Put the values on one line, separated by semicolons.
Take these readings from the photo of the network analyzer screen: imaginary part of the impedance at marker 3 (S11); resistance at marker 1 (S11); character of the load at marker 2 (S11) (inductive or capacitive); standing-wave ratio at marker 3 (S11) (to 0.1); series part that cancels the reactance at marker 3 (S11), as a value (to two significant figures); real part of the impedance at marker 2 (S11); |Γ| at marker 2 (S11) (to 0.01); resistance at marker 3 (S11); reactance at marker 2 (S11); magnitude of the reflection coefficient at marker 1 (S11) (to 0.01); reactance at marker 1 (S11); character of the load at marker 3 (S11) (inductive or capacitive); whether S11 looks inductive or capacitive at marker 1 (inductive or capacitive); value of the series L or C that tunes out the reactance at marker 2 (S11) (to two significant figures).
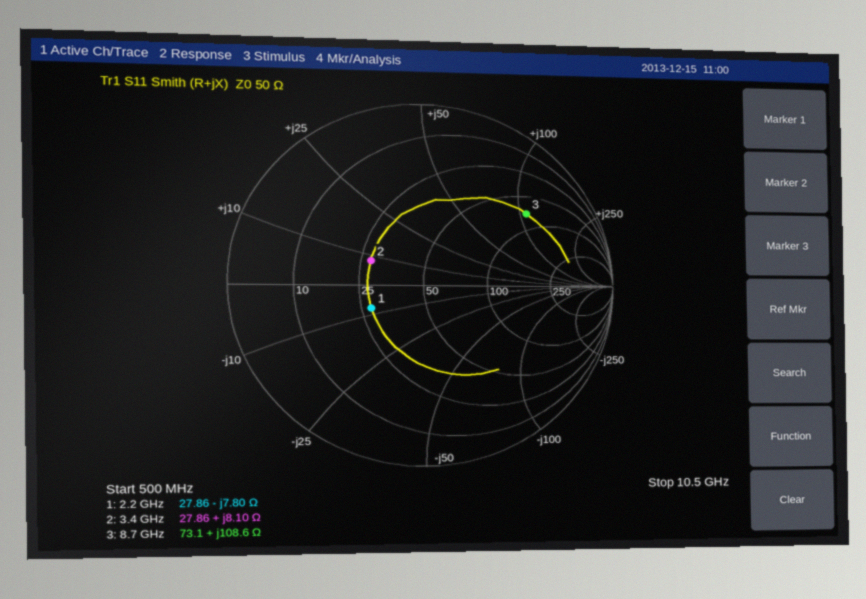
+108.6 Ω; 27.86 Ω; inductive; 5.2; 170 fF; 27.86 Ω; 0.30; 73.1 Ω; +8.10 Ω; 0.30; -7.80 Ω; inductive; capacitive; 5.8 pF
